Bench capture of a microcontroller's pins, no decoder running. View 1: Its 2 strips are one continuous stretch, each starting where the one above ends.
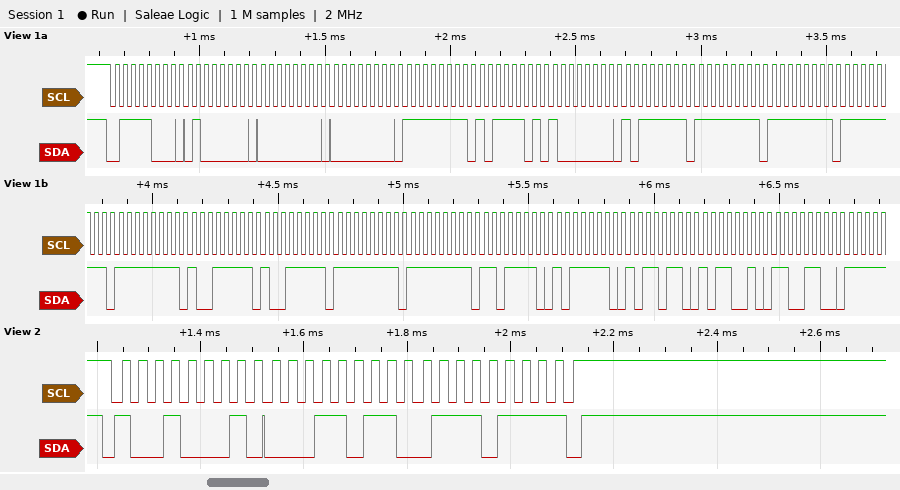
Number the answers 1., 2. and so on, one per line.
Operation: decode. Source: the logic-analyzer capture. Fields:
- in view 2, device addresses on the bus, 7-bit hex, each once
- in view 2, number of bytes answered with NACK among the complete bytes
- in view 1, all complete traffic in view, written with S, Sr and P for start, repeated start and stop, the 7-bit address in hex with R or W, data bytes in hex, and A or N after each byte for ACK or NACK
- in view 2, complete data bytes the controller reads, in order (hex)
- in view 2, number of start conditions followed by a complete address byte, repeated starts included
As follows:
1. 0x48
2. 1
3. S 3CW A 40 A 00 A 00 A FF A BD A 80 A BF A FF A FF A FF A FF A 9F A 9F A FF A FF A DE A BE A B6 A B2 A CC A
4. 1B 77
5. 1
